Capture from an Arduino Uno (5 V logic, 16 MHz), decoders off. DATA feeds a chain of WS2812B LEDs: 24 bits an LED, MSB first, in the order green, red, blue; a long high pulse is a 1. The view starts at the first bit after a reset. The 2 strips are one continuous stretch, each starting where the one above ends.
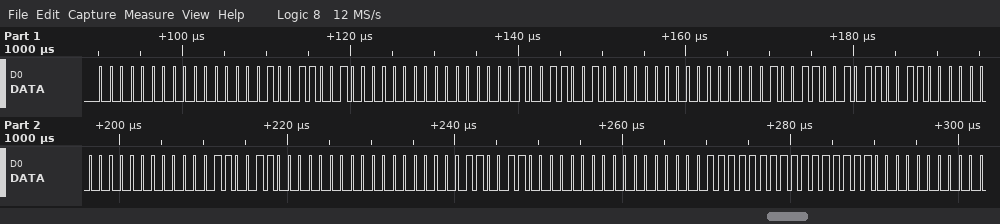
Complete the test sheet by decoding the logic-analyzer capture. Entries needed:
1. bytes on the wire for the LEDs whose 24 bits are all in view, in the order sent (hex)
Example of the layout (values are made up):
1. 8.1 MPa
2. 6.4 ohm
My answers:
1. 00 00 99 00 00 99 00 00 99 66 00 00 66 00 00 66 00 00 FF FF 00
